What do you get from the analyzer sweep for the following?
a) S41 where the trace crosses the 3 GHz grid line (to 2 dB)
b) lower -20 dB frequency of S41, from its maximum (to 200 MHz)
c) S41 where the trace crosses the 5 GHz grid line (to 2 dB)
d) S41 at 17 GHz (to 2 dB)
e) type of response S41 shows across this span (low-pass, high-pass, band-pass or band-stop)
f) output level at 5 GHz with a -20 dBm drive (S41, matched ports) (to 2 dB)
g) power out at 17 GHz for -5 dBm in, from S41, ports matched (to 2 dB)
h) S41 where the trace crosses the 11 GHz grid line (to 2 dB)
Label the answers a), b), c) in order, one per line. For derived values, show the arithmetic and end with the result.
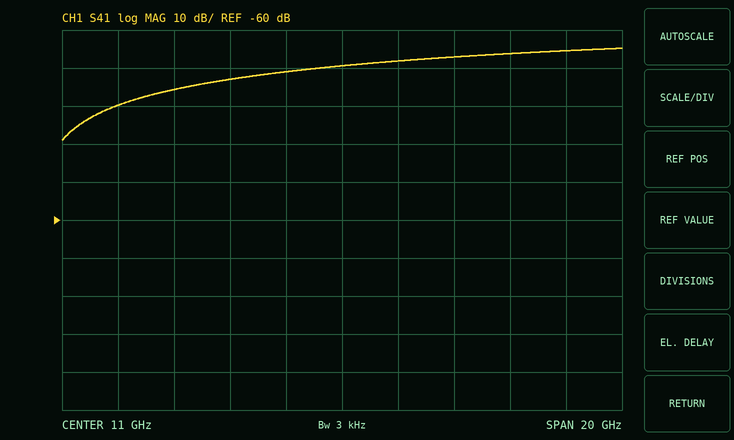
a) -30 dB
b) 1.6 GHz
c) -26 dB
d) -16 dB
e) high-pass
f) -20 dBm + (-26 dB) = -46 dBm
g) -5 dBm + (-16 dB) = -22 dBm
h) -20 dB
